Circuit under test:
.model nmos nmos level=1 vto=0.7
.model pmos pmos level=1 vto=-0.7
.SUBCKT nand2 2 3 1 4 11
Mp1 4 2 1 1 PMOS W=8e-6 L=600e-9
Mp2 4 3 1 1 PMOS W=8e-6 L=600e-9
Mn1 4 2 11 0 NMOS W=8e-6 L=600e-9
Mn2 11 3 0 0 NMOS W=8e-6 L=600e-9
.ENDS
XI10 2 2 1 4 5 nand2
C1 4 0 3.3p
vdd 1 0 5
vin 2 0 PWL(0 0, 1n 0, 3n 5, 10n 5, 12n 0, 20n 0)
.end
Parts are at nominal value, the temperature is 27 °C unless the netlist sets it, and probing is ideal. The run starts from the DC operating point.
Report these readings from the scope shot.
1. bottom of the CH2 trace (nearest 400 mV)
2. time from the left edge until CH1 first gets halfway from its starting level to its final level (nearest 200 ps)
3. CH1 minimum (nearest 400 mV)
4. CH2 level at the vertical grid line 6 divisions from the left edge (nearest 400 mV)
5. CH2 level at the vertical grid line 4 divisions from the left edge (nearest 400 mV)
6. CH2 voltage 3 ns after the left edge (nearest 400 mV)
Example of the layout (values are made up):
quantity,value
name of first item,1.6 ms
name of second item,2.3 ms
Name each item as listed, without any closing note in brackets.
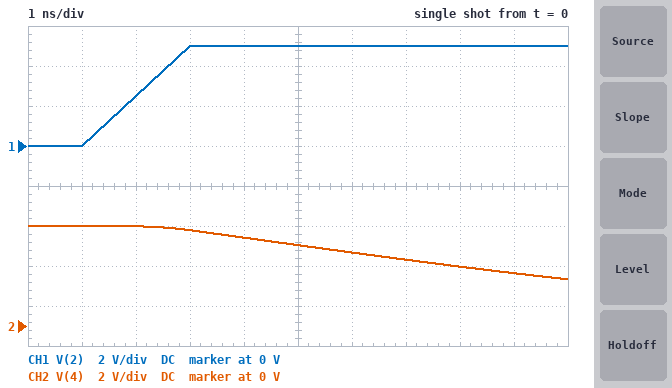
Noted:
quantity,value
bottom of the CH2 trace,2.4 V
time from the left edge until CH1 first gets halfway from its starting level to its final level,2.0 ns
CH1 minimum,0 V
CH2 level at the vertical grid line 6 divisions from the left edge,3.6 V
CH2 level at the vertical grid line 4 divisions from the left edge,4.4 V
CH2 voltage 3 ns after the left edge,4.8 V
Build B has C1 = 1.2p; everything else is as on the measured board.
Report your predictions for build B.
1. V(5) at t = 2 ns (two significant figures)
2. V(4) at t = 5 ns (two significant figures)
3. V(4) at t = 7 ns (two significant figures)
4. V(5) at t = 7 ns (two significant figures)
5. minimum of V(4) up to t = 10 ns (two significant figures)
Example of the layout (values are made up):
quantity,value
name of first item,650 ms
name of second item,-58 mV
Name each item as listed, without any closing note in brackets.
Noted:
quantity,value
V(5) at t = 2 ns,530 mV
V(4) at t = 5 ns,2.5 V
V(4) at t = 7 ns,1.2 V
V(5) at t = 7 ns,540 mV
minimum of V(4) up to t = 10 ns,310 mV
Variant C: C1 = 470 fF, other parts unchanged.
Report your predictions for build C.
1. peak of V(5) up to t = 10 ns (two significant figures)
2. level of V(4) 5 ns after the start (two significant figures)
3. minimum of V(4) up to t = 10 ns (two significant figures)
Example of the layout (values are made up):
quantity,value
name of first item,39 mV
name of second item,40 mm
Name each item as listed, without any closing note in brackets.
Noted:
quantity,value
peak of V(5) up to t = 10 ns,1.2 V
level of V(4) 5 ns after the start,520 mV
minimum of V(4) up to t = 10 ns,1.2 mV
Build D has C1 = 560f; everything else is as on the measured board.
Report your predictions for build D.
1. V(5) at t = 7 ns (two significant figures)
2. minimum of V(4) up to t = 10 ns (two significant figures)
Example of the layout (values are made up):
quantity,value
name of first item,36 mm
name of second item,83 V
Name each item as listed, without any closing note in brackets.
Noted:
quantity,value
V(5) at t = 7 ns,57 mV
minimum of V(4) up to t = 10 ns,5.4 mV
